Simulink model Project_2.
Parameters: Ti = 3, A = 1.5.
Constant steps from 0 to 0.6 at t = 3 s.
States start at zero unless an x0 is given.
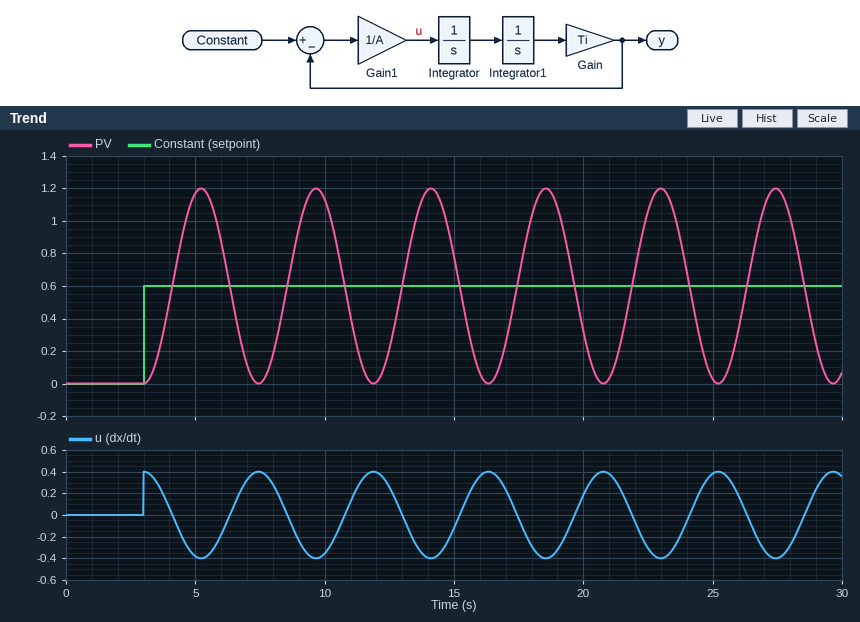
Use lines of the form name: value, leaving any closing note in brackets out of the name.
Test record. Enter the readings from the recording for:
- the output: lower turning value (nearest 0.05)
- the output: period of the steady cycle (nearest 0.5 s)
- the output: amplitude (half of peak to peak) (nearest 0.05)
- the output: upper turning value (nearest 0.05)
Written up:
the output: lower turning value: 0.00
the output: period of the steady cycle: 4.5 s
the output: amplitude (half of peak to peak): 0.60
the output: upper turning value: 1.20
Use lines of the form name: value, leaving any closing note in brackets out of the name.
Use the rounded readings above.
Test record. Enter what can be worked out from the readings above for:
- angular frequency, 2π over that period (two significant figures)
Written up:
angular frequency, 2π over that period: 1.4 rad/s
